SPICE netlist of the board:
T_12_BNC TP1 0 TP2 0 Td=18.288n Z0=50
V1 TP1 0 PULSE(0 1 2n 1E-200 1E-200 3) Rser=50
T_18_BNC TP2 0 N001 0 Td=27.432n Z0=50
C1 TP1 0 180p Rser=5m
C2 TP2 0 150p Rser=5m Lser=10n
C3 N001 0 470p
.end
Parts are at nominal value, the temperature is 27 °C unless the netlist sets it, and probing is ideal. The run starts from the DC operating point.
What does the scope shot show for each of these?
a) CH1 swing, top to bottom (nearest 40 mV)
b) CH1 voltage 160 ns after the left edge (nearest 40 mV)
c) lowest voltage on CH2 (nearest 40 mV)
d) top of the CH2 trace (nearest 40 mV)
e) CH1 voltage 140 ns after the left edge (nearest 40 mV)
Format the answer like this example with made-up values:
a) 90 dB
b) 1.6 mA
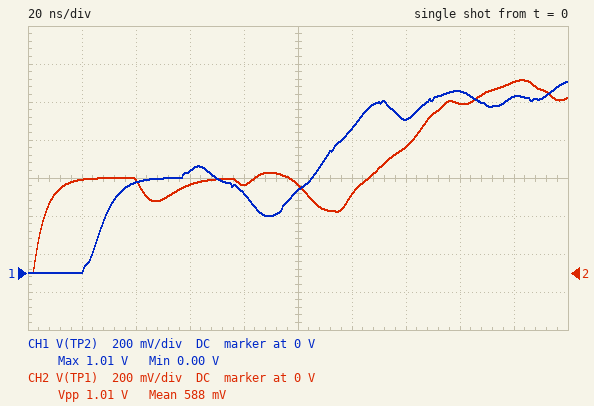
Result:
a) 1.00 V
b) 960 mV
c) 0 V
d) 1.00 V
e) 800 mV
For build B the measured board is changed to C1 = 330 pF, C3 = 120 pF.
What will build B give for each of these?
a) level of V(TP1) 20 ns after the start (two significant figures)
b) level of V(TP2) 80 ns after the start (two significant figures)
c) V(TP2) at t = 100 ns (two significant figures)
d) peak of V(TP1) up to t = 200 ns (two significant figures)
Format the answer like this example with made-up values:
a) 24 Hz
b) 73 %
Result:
a) 440 mV
b) 460 mV
c) 750 mV
d) 1.0 V
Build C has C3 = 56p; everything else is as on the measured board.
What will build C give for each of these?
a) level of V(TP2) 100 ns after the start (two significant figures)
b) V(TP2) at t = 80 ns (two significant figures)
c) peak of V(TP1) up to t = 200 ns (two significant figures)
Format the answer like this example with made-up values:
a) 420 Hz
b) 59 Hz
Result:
a) 930 mV
b) 470 mV
c) 1.1 V
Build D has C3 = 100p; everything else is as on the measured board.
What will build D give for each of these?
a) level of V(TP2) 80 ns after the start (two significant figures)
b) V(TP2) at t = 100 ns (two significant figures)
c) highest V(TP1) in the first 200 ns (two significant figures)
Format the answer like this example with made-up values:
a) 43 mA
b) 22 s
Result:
a) 450 mV
b) 860 mV
c) 1.1 V
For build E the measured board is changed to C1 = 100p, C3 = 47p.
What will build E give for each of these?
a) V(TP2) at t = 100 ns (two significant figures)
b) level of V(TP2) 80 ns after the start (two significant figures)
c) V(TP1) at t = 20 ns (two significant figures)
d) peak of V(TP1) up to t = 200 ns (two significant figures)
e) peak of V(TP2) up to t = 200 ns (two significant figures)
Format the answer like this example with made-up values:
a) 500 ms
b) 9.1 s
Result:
a) 960 mV
b) 490 mV
c) 500 mV
d) 1.1 V
e) 1.0 V
